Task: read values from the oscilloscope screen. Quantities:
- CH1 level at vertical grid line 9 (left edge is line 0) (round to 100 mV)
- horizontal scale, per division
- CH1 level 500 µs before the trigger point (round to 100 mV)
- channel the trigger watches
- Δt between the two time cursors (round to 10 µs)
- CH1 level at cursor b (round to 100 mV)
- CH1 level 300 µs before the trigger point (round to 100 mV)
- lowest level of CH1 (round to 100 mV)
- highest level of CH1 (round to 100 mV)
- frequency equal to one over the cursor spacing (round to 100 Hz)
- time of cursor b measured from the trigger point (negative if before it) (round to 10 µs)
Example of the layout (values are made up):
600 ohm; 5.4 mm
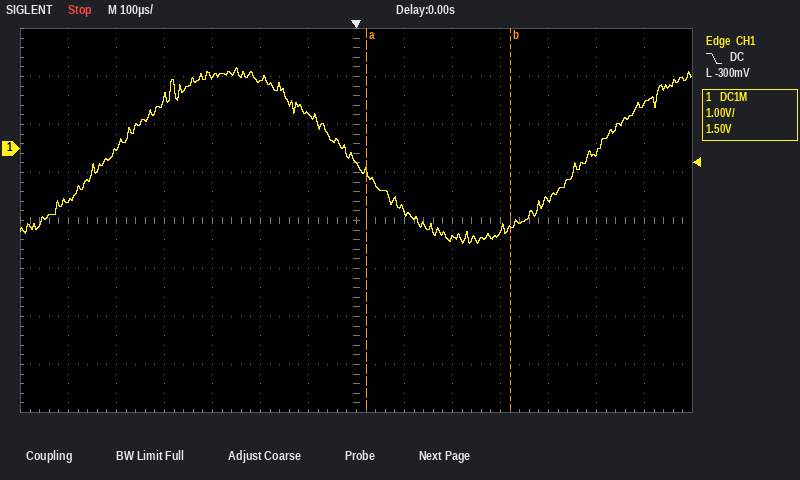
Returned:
-1.9 V; 100 µs; 0.0 V; CH1; 300 µs; -1.7 V; 1.5 V; -2.0 V; 1.7 V; 3.3 kHz; +320 µs
